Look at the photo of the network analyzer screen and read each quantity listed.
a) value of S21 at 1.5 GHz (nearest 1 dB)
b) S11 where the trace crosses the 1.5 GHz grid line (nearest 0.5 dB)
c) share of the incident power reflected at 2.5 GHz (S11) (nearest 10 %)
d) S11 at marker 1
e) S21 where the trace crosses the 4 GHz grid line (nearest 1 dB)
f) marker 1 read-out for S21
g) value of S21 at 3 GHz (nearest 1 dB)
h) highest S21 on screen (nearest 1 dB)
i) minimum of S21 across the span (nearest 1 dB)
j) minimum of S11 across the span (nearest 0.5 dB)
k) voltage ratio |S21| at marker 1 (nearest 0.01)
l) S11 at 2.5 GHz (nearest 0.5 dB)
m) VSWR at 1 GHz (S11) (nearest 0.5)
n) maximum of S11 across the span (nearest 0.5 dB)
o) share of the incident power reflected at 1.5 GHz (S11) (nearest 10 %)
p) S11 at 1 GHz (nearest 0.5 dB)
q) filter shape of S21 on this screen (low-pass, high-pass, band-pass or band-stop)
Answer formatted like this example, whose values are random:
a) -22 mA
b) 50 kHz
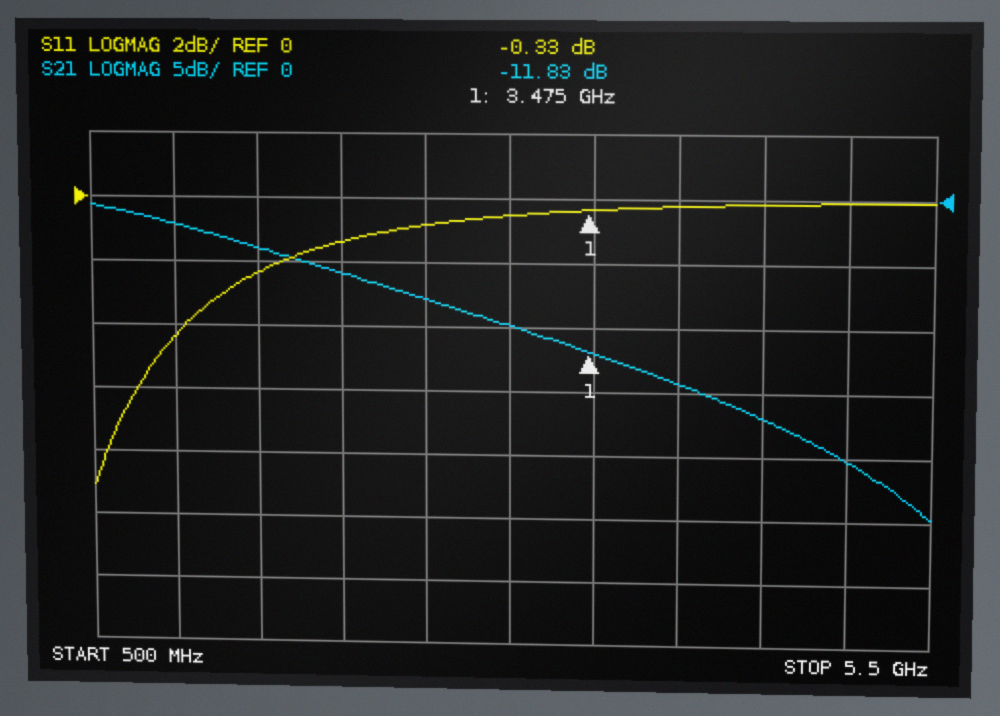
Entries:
a) -4 dB
b) -2.5 dB
c) 80 %
d) -0.33 dB
e) -14 dB
f) -11.83 dB
g) -10 dB
h) -1 dB
i) -25 dB
j) -9.0 dB
k) 0.26
l) -1.0 dB
m) 4.0
n) 0.0 dB
o) 60 %
p) -4.5 dB
q) low-pass
